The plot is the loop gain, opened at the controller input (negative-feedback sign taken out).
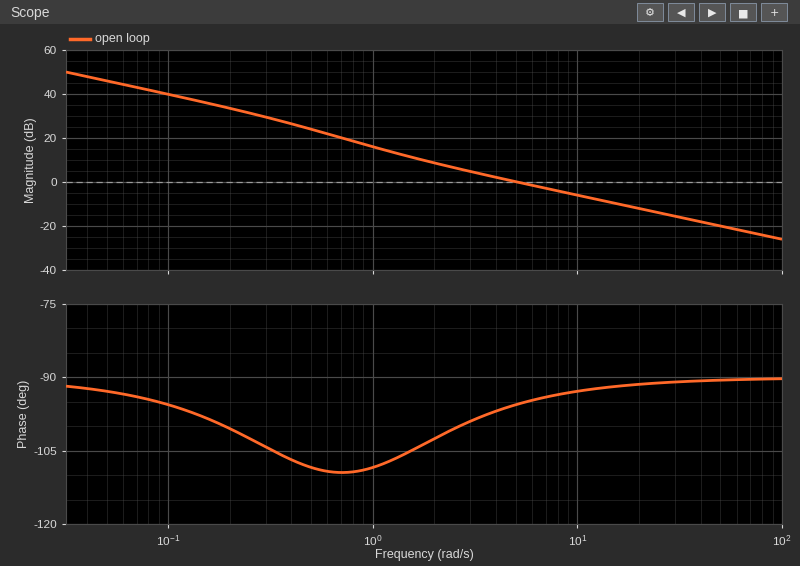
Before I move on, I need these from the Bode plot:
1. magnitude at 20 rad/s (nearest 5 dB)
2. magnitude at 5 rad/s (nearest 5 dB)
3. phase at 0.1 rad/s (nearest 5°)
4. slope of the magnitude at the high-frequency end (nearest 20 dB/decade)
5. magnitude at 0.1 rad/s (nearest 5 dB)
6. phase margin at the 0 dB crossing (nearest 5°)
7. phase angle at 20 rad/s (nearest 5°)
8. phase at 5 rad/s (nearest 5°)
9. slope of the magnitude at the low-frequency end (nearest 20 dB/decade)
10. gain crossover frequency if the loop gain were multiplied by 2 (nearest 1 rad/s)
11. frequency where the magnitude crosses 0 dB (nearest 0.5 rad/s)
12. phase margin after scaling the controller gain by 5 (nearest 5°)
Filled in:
-10 dB
0 dB
-95°
-20 dB/decade
40 dB
85°
-90°
-95°
-20 dB/decade
10 rad/s
5.0 rad/s
90°
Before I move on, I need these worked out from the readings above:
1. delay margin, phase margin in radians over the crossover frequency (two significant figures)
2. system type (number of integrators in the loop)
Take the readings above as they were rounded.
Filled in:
0.30 s
1
